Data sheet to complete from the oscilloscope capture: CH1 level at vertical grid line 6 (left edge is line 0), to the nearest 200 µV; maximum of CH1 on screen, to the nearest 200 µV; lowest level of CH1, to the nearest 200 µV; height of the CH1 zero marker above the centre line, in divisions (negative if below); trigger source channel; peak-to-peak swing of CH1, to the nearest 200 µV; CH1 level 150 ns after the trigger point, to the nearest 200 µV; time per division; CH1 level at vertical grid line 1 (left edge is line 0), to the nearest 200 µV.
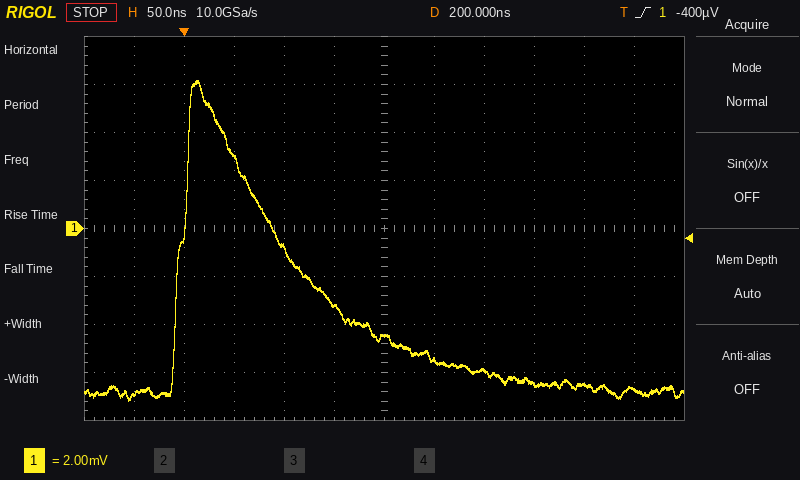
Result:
-4.4 mV
6.2 mV
-7.2 mV
0.0 div
CH1
13.4 mV
-3.2 mV
50 ns
-6.8 mV
